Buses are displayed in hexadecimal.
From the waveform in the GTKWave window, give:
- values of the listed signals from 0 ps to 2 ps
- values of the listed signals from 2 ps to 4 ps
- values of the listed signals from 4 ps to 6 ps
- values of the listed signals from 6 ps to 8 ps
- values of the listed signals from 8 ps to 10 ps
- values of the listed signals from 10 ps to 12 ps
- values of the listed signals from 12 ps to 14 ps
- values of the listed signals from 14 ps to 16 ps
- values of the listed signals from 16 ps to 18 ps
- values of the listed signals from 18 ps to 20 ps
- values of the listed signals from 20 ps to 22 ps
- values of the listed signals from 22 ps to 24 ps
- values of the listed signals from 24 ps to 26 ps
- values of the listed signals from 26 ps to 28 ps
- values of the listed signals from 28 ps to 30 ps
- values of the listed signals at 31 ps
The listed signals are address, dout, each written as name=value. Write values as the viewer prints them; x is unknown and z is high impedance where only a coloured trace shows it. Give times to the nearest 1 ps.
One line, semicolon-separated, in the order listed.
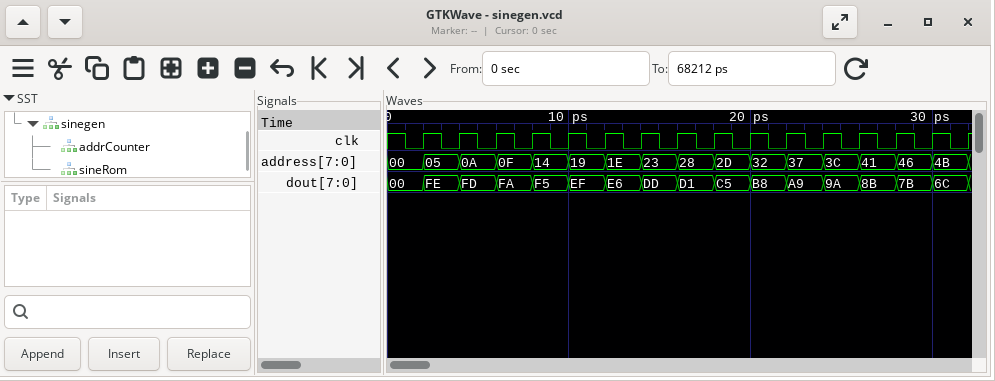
address=00, dout=00; address=05, dout=FE; address=0A, dout=FD; address=0F, dout=FA; address=14, dout=F5; address=19, dout=EF; address=1E, dout=E6; address=23, dout=DD; address=28, dout=D1; address=2D, dout=C5; address=32, dout=B8; address=37, dout=A9; address=3C, dout=9A; address=41, dout=8B; address=46, dout=7B; address=4B, dout=6C
